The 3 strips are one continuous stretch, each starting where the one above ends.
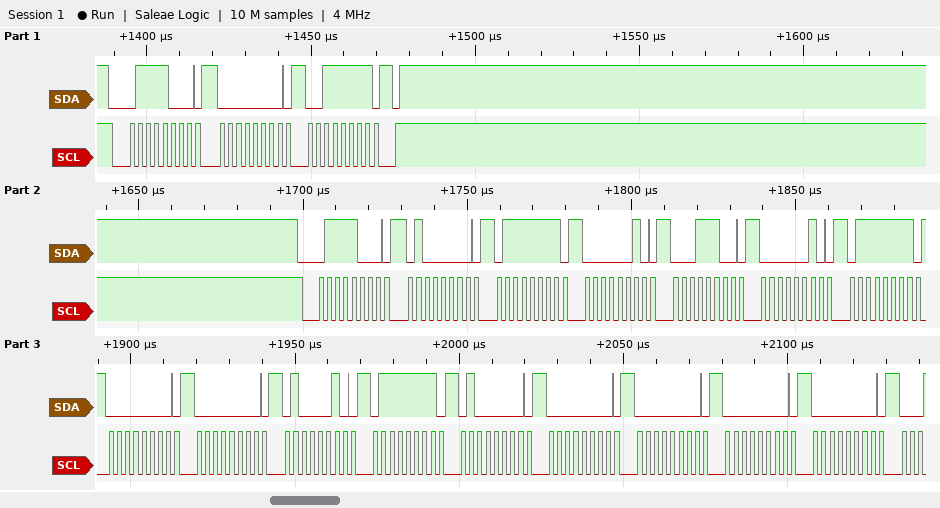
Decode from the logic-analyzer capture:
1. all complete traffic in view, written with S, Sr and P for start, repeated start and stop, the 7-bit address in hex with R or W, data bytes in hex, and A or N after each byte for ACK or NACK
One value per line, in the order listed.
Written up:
S 3CW A 00 A 3F A P S 3CW A 40 A 7F A 02 A 1C A 02 A 7F A 00 A 00 A 42 A 7F A 40 A 00 A 00 A 00 A 00 A
